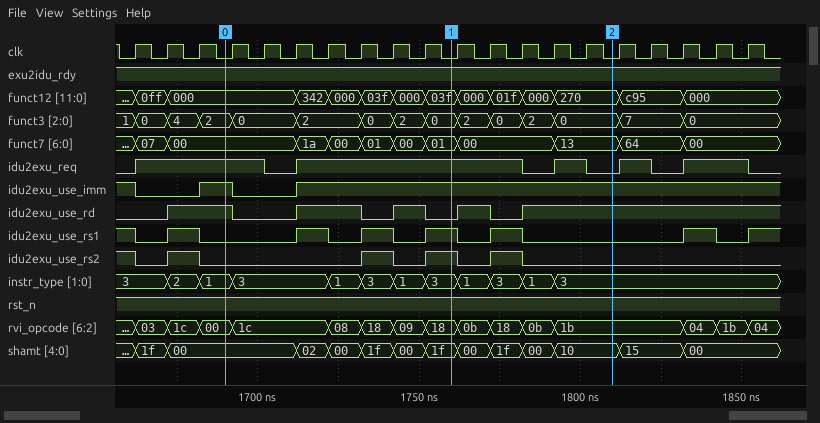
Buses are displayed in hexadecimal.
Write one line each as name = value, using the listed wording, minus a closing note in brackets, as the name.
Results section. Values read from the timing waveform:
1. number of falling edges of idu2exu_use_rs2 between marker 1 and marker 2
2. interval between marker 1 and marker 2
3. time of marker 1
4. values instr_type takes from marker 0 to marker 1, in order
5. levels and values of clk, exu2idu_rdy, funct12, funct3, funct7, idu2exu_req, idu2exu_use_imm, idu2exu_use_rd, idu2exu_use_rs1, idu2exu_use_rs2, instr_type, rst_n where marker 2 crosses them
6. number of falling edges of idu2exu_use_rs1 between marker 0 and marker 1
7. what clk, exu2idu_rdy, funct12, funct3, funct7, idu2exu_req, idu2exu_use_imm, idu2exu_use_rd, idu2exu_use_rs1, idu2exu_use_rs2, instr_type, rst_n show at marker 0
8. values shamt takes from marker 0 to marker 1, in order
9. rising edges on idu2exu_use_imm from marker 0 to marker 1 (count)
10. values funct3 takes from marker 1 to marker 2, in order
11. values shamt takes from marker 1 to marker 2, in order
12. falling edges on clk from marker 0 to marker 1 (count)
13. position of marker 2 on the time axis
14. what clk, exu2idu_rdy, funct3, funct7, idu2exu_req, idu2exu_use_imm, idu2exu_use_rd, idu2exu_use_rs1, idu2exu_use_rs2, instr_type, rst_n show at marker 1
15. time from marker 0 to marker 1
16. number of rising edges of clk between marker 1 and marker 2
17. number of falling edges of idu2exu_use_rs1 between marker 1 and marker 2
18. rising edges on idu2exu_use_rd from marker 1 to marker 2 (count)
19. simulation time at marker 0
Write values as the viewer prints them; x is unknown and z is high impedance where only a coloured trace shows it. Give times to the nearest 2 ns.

number of falling edges of idu2exu_use_rs2 between marker 1 and marker 2 = 2
interval between marker 1 and marker 2 = 50 ns
time of marker 1 = 1760 ns
values instr_type takes from marker 0 to marker 1, in order = 1, 3, 1, 3, 1, 3
levels and values of clk, exu2idu_rdy, funct12, funct3, funct7, idu2exu_req, idu2exu_use_imm, idu2exu_use_rd, idu2exu_use_rs1, idu2exu_use_rs2, instr_type, rst_n where marker 2 crosses them = clk=0, exu2idu_rdy=1, funct12=270, funct3=0, funct7=13, idu2exu_req=0, idu2exu_use_imm=1, idu2exu_use_rd=1, idu2exu_use_rs1=0, idu2exu_use_rs2=0, instr_type=3, rst_n=1
number of falling edges of idu2exu_use_rs1 between marker 0 and marker 1 = 2
what clk, exu2idu_rdy, funct12, funct3, funct7, idu2exu_req, idu2exu_use_imm, idu2exu_use_rd, idu2exu_use_rs1, idu2exu_use_rs2, instr_type, rst_n show at marker 0 = clk=0, exu2idu_rdy=1, funct12=000, funct3=2, funct7=00, idu2exu_req=1, idu2exu_use_imm=1, idu2exu_use_rd=1, idu2exu_use_rs1=0, idu2exu_use_rs2=0, instr_type=1, rst_n=1
values shamt takes from marker 0 to marker 1, in order = 00, 02, 00, 1f, 00, 1f
rising edges on idu2exu_use_imm from marker 0 to marker 1 = 1
values funct3 takes from marker 1 to marker 2, in order = 0, 2, 0, 2, 0
values shamt takes from marker 1 to marker 2, in order = 1f, 00, 1f, 00, 10
falling edges on clk from marker 0 to marker 1 = 7
position of marker 2 on the time axis = 1810 ns
what clk, exu2idu_rdy, funct3, funct7, idu2exu_req, idu2exu_use_imm, idu2exu_use_rd, idu2exu_use_rs1, idu2exu_use_rs2, instr_type, rst_n show at marker 1 = clk=0, exu2idu_rdy=1, funct3=0, funct7=01, idu2exu_req=1, idu2exu_use_imm=1, idu2exu_use_rd=0, idu2exu_use_rs1=1, idu2exu_use_rs2=1, instr_type=3, rst_n=1
time from marker 0 to marker 1 = 70 ns
number of rising edges of clk between marker 1 and marker 2 = 5
number of falling edges of idu2exu_use_rs1 between marker 1 and marker 2 = 2
rising edges on idu2exu_use_rd from marker 1 to marker 2 = 2
simulation time at marker 0 = 1690 ns
